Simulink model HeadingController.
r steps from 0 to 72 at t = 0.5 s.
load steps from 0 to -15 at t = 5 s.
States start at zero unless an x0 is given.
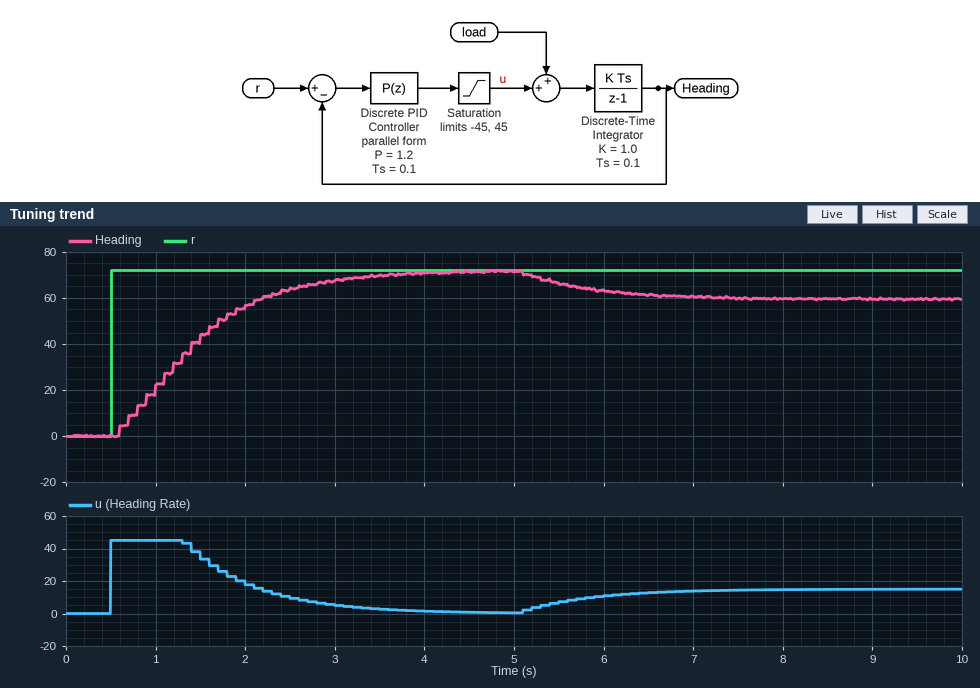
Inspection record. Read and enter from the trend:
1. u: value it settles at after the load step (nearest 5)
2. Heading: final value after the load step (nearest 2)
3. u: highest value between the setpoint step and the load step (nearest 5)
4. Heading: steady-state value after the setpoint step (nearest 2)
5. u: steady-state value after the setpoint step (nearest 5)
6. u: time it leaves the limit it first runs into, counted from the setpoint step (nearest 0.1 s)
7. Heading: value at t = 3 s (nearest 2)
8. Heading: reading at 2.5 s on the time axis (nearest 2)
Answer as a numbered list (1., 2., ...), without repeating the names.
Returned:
1. 15
2. 60
3. 45
4. 72
5. 0
6. 0.8 s
7. 68
8. 64
